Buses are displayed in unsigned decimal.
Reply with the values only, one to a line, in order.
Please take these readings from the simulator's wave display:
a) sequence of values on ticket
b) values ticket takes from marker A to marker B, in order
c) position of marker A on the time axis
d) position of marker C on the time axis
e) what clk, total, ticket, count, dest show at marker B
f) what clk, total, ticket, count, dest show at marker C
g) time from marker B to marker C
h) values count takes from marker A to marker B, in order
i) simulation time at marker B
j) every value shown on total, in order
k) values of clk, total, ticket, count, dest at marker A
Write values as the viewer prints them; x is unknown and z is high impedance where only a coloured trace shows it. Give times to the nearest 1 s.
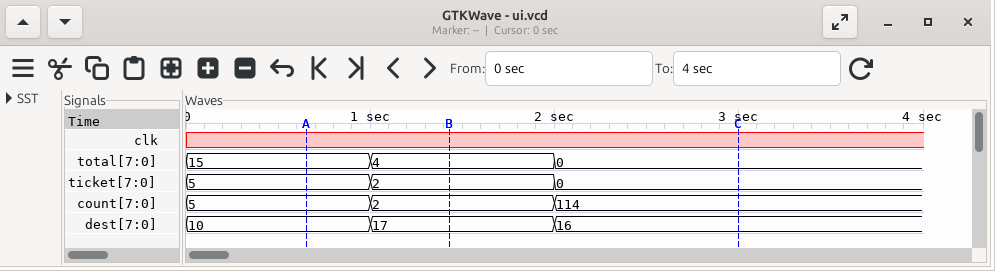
5, 2, 0
5, 2
1 s
3 s
clk=x, total=4, ticket=2, count=2, dest=17
clk=x, total=0, ticket=0, count=114, dest=16
2 s
5, 2
1 s
15, 4, 0
clk=x, total=15, ticket=5, count=5, dest=10
